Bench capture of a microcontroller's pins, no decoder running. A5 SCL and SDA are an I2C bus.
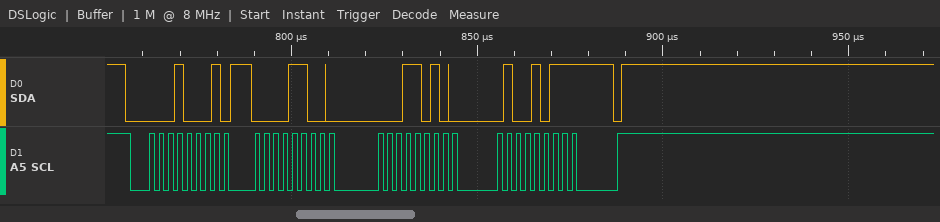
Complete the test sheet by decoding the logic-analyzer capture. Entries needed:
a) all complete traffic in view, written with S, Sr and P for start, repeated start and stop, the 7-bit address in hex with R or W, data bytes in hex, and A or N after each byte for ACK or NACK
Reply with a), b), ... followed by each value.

a) S 08R A 0C A 1A A 4B N P
